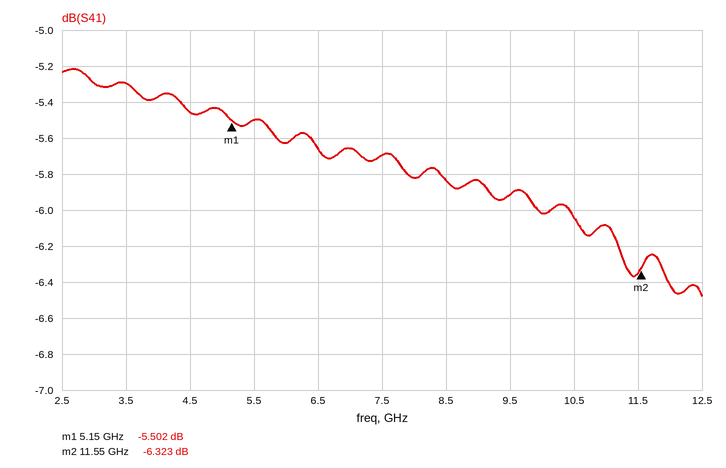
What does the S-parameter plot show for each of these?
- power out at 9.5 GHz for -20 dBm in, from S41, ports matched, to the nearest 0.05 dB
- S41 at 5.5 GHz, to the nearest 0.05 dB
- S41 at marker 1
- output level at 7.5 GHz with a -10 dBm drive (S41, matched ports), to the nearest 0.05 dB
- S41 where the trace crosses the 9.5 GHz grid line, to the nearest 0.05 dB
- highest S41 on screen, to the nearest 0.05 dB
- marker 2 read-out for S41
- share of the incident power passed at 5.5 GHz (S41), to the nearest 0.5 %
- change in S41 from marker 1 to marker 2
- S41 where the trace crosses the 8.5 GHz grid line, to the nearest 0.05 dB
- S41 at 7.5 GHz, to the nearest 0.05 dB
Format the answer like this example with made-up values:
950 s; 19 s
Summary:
-25.90 dBm; -5.50 dB; -5.502 dB; -15.70 dBm; -5.90 dB; -5.20 dB; -6.323 dB; 28.0 %; -0.821 dB; -5.85 dB; -5.70 dB
